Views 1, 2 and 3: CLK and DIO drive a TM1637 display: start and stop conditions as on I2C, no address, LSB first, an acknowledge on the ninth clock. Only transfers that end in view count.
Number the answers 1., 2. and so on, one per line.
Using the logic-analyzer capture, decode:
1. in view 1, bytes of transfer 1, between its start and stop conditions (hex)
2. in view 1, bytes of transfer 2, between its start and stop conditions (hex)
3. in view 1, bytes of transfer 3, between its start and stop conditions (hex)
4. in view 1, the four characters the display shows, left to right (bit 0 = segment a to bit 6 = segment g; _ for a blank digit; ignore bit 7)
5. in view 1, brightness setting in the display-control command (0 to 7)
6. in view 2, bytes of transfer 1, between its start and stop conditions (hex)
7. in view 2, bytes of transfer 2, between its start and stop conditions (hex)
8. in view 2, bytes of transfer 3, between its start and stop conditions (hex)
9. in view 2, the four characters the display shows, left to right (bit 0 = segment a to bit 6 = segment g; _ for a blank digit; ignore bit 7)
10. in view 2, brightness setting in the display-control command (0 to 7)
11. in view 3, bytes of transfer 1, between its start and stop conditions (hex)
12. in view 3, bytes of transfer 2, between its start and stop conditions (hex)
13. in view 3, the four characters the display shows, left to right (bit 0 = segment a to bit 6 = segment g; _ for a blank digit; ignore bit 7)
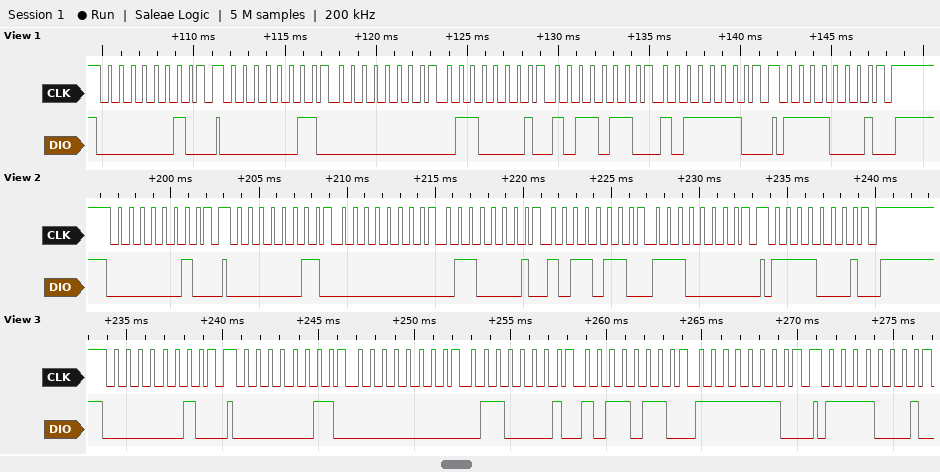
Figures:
1. 40
2. C0 00 86 6D 7D
3. 8F
4. _156
5. 7
6. 40
7. C0 00 86 6D 07
8. 8F
9. _157
10. 7
11. 40
12. C0 00 86 6D 7F
13. _158
